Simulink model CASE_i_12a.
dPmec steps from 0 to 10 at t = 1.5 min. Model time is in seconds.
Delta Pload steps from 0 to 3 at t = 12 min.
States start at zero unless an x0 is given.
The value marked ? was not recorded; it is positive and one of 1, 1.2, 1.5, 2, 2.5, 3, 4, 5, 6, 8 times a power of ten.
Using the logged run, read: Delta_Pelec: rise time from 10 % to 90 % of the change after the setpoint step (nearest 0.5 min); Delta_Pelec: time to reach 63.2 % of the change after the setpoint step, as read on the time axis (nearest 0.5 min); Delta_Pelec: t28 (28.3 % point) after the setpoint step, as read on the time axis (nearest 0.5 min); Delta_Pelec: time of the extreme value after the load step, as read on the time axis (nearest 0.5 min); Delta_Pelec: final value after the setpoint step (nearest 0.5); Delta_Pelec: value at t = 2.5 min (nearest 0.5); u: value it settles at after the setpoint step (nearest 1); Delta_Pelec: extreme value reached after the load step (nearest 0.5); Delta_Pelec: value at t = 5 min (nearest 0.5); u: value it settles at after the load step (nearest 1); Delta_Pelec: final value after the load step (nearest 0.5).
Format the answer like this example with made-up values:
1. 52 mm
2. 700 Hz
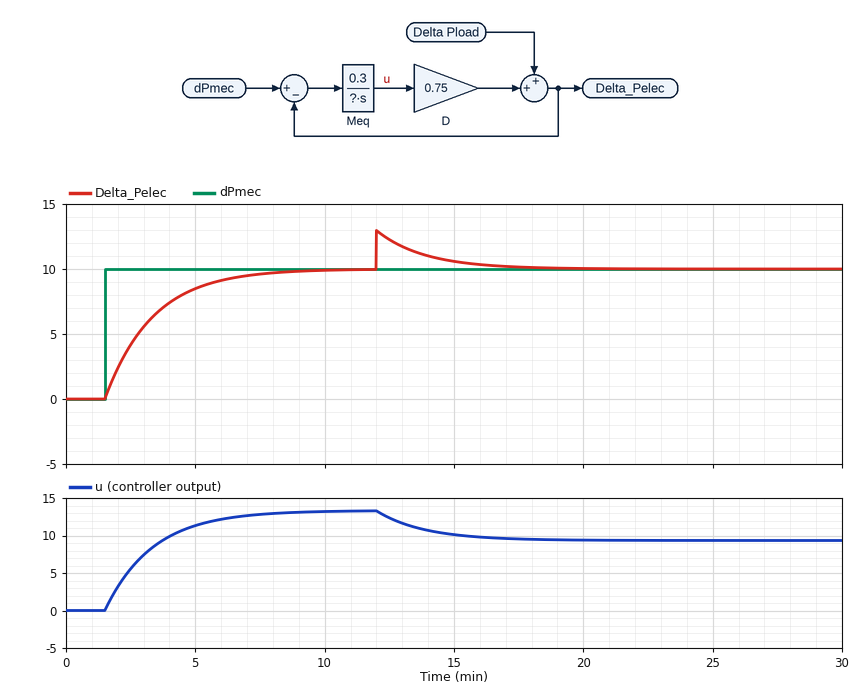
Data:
1. 4.0 min
2. 3.5 min
3. 2.0 min
4. 12.0 min
5. 10.0
6. 4.0
7. 13
8. 13.0
9. 8.5
10. 9
11. 10.0
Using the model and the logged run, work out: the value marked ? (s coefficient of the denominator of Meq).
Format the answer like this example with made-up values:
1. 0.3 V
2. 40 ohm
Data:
1. 25
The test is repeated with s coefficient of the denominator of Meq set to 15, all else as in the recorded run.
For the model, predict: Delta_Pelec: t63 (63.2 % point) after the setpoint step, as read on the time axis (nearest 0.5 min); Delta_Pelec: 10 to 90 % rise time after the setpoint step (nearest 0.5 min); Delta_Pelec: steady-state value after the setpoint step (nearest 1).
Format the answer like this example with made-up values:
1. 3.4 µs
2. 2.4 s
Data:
1. 2.5 min
2. 2.5 min
3. 10
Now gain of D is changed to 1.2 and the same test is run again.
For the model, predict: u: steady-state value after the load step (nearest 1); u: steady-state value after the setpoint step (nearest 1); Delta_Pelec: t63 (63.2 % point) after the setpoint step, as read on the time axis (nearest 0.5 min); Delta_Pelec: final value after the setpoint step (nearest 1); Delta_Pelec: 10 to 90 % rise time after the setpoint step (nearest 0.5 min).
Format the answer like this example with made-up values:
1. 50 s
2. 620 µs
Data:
1. 6
2. 8
3. 2.5 min
4. 10
5. 2.5 min
